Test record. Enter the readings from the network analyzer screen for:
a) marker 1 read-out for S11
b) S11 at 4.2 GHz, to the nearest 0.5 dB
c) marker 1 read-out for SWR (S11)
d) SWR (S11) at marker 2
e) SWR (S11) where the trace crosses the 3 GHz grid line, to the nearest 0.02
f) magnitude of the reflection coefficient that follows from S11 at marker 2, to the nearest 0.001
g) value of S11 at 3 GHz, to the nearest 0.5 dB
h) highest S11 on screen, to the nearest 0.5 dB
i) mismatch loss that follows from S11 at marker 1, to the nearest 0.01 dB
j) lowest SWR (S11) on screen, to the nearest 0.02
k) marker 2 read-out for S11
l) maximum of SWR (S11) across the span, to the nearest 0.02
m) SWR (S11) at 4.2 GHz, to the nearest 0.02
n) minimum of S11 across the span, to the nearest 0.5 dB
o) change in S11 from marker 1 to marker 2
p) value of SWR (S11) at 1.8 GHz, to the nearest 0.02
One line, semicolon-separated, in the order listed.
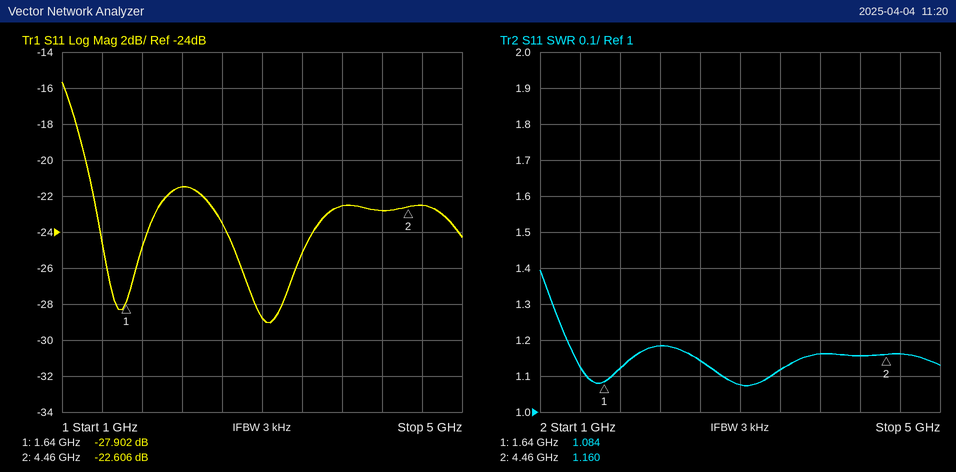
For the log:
-27.902 dB; -23.0 dB; 1.084; 1.160; 1.08; 0.074; -29.0 dB; -15.5 dB; 0.01 dB; 1.08; -22.606 dB; 1.40; 1.16; -29.0 dB; 5.296 dB; 1.12
